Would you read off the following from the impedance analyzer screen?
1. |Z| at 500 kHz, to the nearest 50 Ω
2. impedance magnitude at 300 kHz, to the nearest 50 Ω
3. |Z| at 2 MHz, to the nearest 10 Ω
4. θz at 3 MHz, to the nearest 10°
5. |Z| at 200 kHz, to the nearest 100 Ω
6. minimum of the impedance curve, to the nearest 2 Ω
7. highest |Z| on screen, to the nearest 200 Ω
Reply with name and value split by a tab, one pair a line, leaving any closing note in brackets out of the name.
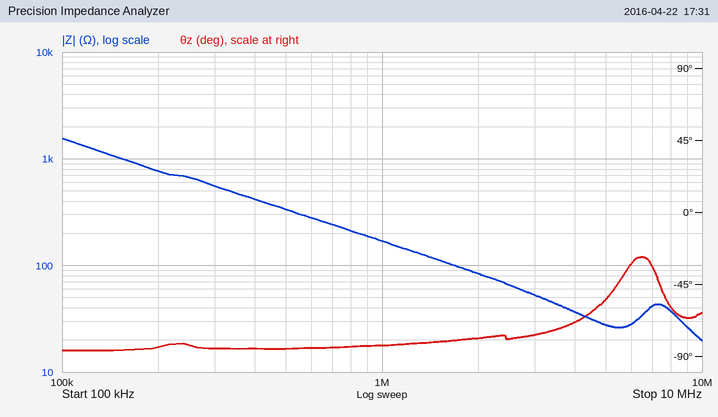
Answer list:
|Z| at 500 kHz, to the nearest 50 Ω	350 Ω
impedance magnitude at 300 kHz, to the nearest 50 Ω	550 Ω
|Z| at 2 MHz, to the nearest 10 Ω	80 Ω
θz at 3 MHz, to the nearest 10°	-80°
|Z| at 200 kHz, to the nearest 100 Ω	800 Ω
minimum of the impedance curve, to the nearest 2 Ω	20 Ω
highest |Z| on screen, to the nearest 200 Ω	1.6 kΩ
